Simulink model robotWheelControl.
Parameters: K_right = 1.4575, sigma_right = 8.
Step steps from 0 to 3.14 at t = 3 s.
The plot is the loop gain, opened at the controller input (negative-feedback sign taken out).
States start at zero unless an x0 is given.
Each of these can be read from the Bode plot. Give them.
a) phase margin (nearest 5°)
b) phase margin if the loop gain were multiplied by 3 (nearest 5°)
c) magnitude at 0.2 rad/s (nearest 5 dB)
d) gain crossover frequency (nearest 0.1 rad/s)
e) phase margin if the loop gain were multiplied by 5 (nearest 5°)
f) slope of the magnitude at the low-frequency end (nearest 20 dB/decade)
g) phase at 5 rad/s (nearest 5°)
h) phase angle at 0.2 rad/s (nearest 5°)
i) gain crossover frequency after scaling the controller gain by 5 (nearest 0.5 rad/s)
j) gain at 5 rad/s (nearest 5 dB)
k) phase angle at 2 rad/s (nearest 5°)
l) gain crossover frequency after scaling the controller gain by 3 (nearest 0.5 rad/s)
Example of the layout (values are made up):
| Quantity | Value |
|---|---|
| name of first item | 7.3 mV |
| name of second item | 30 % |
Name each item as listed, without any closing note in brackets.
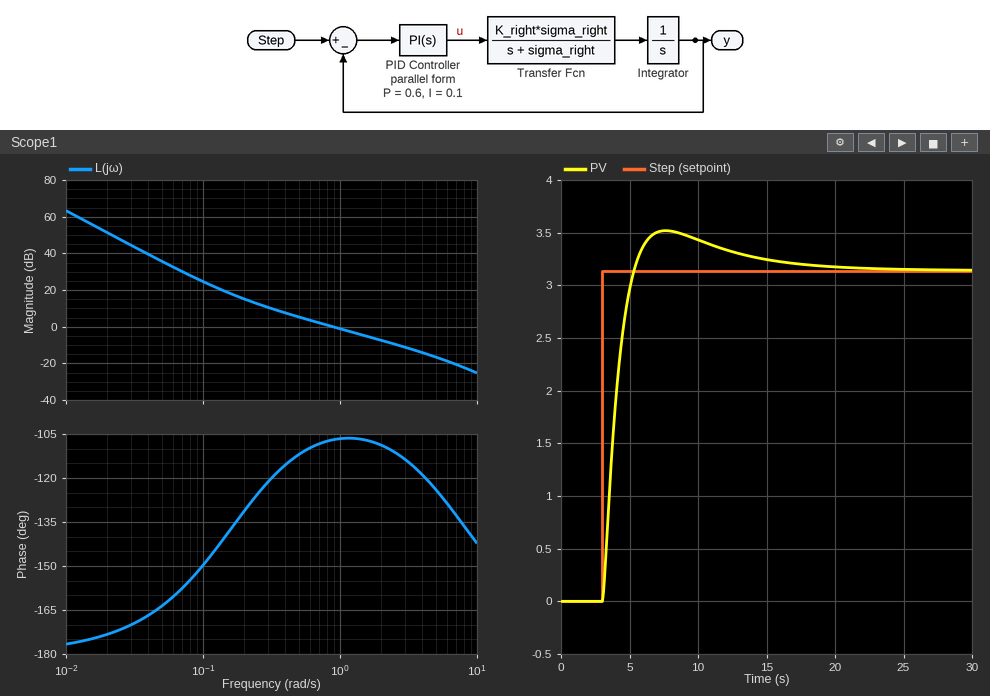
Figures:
| Quantity | Value |
|---|---|
| phase margin | 75° |
| phase margin if the loop gain were multiplied by 3 | 70° |
| magnitude at 0.2 rad/s | 15 dB |
| gain crossover frequency | 0.9 rad/s |
| phase margin if the loop gain were multiplied by 5 | 60° |
| slope of the magnitude at the low-frequency end | -40 dB/decade |
| phase at 5 rad/s | -125° |
| phase angle at 0.2 rad/s | -130° |
| gain crossover frequency after scaling the controller gain by 5 | 4.0 rad/s |
| gain at 5 rad/s | -15 dB |
| phase angle at 2 rad/s | -110° |
| gain crossover frequency after scaling the controller gain by 3 | 2.5 rad/s |
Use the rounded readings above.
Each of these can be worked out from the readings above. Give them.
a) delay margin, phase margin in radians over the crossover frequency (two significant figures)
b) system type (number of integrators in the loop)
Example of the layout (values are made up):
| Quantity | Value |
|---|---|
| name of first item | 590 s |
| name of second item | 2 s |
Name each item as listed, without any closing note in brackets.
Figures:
| Quantity | Value |
|---|---|
| delay margin, phase margin in radians over the crossover frequency | 1.5 s |
| system type | 2 |
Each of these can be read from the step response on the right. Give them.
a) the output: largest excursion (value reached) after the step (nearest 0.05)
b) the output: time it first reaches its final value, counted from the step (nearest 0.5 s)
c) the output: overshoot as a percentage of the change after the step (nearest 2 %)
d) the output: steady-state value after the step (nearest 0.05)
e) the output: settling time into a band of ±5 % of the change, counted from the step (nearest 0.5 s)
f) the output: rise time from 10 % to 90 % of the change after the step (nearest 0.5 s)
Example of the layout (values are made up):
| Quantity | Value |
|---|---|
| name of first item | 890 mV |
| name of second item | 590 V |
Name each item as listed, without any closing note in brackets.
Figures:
| Quantity | Value |
|---|---|
| the output: largest excursion (value reached) after the step | 3.50 |
| the output: time it first reaches its final value, counted from the step | 2.5 s |
| the output: overshoot as a percentage of the change after the step | 12 % |
| the output: steady-state value after the step | 3.15 |
| the output: settling time into a band of ±5 % of the change, counted from the step | 10.0 s |
| the output: rise time from 10 % to 90 % of the change after the step | 1.5 s |
